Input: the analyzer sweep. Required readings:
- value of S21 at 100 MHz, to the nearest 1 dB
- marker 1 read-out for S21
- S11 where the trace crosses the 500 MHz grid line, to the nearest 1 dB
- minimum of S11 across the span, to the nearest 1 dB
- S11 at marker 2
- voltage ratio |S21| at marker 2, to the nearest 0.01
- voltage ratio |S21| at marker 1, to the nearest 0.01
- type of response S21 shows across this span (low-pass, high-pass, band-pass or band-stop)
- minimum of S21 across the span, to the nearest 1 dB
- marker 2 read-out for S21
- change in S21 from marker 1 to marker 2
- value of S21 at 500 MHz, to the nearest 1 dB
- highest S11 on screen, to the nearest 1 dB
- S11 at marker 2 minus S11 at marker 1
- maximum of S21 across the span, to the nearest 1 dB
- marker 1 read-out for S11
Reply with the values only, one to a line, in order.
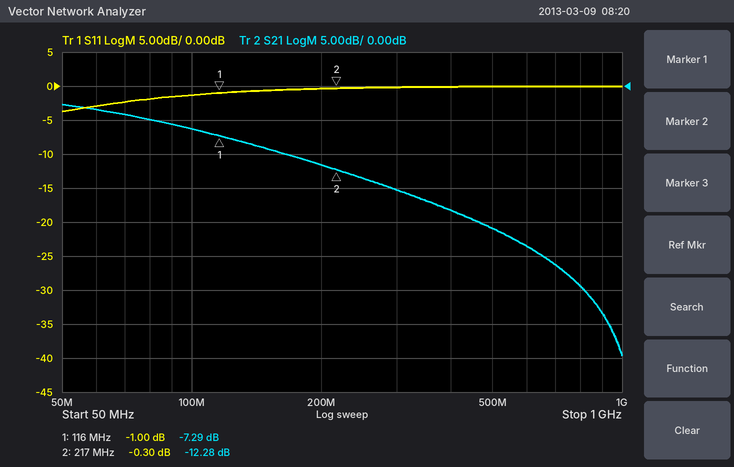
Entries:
-6 dB
-7.29 dB
0 dB
-4 dB
-0.30 dB
0.24
0.43
low-pass
-40 dB
-12.28 dB
-4.99 dB
-21 dB
0 dB
0.70 dB
-3 dB
-1.00 dB
